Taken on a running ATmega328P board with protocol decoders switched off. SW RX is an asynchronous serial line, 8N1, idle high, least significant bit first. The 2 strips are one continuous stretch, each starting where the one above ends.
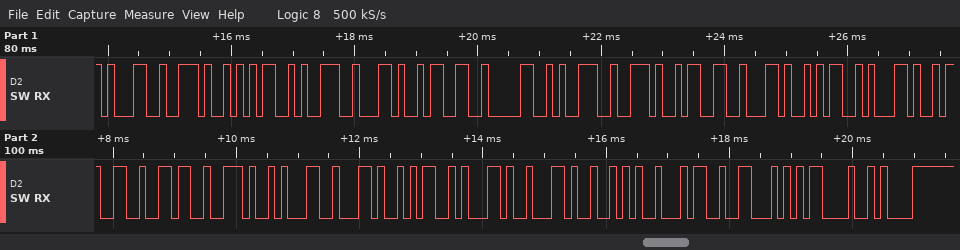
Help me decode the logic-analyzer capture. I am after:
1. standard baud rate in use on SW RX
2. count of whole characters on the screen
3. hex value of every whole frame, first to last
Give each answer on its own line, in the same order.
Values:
9600 baud
26
31 2E 35 39 2C 33 30 39 2E 33 2C 4D 2C 33 36 2E 31 2C 4D 2C 2C 2A 34 46 0D 0A
